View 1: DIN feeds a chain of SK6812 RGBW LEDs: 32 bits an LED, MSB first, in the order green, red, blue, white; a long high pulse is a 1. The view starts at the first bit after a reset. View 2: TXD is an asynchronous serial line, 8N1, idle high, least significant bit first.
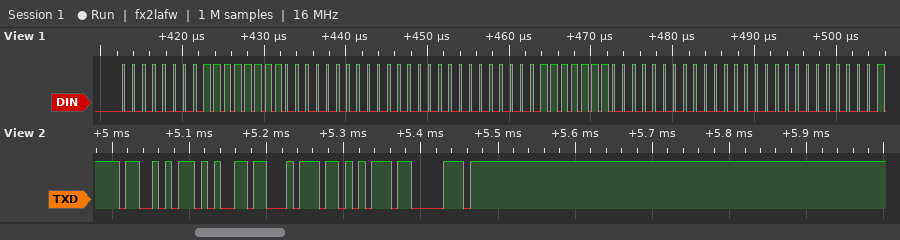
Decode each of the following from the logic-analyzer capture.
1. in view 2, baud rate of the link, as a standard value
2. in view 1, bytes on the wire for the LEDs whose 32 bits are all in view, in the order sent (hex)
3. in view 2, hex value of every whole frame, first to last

115200 baud
00 FF 00 00 00 7F 00 00
0x53 0x65 0x74 0x75 0x70
